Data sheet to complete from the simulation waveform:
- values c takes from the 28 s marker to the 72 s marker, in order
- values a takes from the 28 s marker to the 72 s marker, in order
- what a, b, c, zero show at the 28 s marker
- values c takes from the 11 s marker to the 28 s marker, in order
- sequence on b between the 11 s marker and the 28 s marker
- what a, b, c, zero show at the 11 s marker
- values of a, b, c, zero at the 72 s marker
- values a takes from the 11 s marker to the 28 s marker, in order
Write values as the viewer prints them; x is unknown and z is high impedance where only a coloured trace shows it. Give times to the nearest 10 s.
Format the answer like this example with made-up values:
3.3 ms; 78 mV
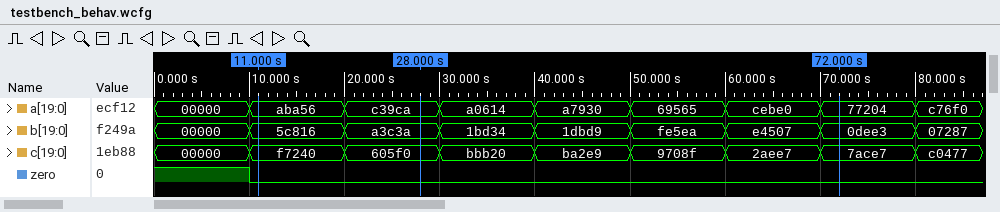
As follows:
605f0, bbb20, ba2e9, 9708f, 2aee7, 7ace7; c39ca, a0614, a7930, 69565, cebe0, 77204; a=c39ca, b=a3c3a, c=605f0, zero=0; f7240, 605f0; 5c816, a3c3a; a=aba56, b=5c816, c=f7240, zero=0; a=77204, b=0dee3, c=7ace7, zero=0; aba56, c39ca
